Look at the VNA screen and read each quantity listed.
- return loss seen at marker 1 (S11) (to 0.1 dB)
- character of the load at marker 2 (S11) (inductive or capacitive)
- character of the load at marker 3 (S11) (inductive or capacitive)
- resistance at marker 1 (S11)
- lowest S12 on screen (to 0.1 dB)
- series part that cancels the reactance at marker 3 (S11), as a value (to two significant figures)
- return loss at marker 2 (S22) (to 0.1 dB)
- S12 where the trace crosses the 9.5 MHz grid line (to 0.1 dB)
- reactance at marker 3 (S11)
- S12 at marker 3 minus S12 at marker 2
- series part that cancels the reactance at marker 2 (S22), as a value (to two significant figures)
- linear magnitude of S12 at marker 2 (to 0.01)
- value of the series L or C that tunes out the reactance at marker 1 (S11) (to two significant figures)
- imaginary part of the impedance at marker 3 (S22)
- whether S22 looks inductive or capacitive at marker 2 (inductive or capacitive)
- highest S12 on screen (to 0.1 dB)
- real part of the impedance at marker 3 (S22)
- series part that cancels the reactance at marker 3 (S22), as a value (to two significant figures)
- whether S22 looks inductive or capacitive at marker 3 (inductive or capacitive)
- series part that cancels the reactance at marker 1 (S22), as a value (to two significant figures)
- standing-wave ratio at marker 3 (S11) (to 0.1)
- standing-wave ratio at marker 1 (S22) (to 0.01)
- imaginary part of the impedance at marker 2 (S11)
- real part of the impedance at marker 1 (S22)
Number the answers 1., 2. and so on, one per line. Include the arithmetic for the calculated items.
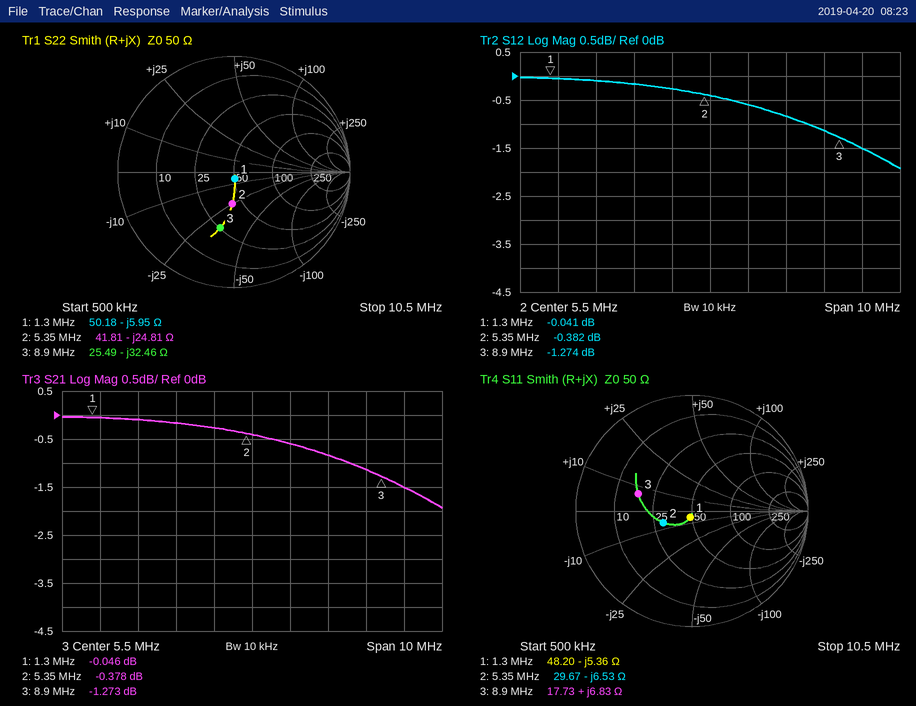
1. 24.8 dB
2. capacitive
3. inductive
4. 48.20 Ω
5. -1.9 dB
6. C = 1/(2π × 8.9 MHz × 6.83 Ω) ≈ 2.6 nF
7. 11.2 dB
8. -1.5 dB
9. +6.83 Ω
10. -1.274 − (-0.382) = -0.892 dB
11. L = 24.81 Ω/(2π × 5.35 MHz) ≈ 738 nH, so 740 nH to two significant figures
12. 10^(-0.382/20) ≈ 0.96
13. L = 5.36 Ω/(2π × 1.3 MHz) ≈ 656 nH, so 660 nH to two significant figures
14. -32.46 Ω
15. capacitive
16. 0.0 dB
17. 25.49 Ω
18. L = 32.46 Ω/(2π × 8.9 MHz) ≈ 580 nH
19. capacitive
20. L = 5.95 Ω/(2π × 1.3 MHz) ≈ 728 nH, so 730 nH to two significant figures
21. 2.9
22. 1.13
23. -6.53 Ω
24. 50.18 Ω
